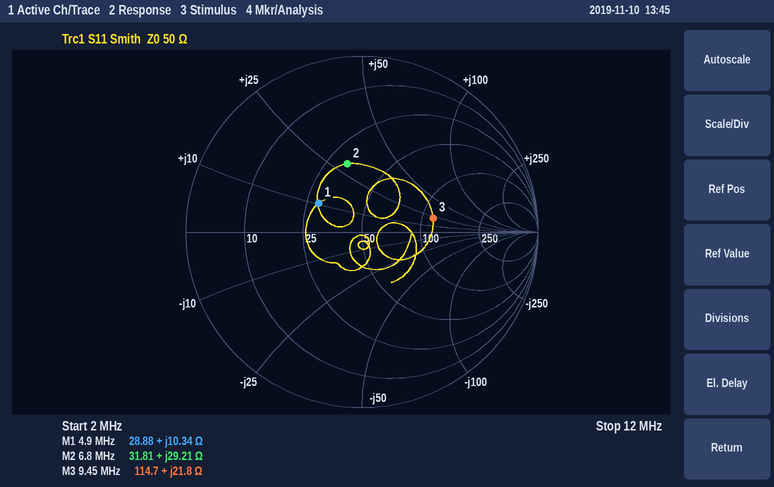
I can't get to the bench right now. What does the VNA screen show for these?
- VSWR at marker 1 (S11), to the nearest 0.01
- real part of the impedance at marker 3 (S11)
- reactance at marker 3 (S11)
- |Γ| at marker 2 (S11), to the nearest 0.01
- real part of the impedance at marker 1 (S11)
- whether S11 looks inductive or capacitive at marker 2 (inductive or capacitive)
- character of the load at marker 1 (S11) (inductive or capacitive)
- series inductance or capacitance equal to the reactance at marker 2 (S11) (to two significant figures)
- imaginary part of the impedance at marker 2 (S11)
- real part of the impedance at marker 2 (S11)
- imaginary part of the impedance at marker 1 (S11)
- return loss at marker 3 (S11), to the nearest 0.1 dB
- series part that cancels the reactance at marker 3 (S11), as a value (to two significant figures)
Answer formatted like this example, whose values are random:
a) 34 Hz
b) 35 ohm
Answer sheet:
a) 1.84
b) 114.7 Ω
c) +21.8 Ω
d) 0.40
e) 28.88 Ω
f) inductive
g) inductive
h) 680 nH
i) +29.21 Ω
j) 31.81 Ω
k) +10.34 Ω
l) 7.7 dB
m) 770 pF
